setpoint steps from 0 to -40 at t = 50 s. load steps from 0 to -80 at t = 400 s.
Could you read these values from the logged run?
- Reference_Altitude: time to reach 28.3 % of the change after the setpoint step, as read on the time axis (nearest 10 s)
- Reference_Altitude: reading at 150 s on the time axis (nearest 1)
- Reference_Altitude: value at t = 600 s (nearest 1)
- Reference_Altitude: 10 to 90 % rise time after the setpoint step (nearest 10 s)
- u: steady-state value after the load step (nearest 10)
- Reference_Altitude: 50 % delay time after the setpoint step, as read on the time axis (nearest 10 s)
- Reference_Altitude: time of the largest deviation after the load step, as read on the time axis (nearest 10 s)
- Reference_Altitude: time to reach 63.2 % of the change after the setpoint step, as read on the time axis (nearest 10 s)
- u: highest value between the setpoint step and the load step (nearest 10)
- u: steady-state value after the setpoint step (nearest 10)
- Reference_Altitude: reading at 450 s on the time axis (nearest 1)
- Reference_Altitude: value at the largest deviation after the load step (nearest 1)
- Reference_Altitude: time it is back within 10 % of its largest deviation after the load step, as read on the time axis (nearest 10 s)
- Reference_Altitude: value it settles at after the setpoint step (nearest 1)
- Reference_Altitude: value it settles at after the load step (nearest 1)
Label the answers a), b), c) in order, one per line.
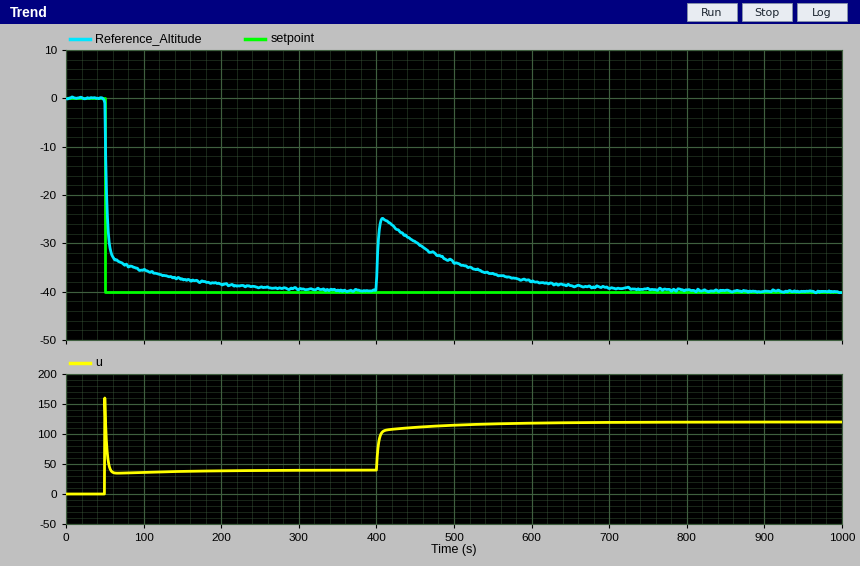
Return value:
a) 50 s
b) -37
c) -38
d) 60 s
e) 120
f) 50 s
g) 410 s
h) 50 s
i) 160
j) 40
k) -30
l) -25
m) 640 s
n) -40
o) -40
